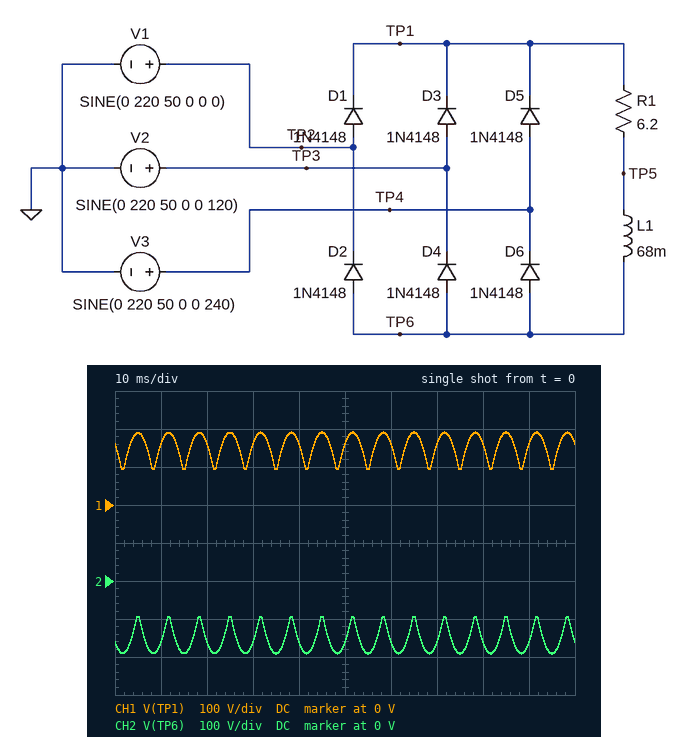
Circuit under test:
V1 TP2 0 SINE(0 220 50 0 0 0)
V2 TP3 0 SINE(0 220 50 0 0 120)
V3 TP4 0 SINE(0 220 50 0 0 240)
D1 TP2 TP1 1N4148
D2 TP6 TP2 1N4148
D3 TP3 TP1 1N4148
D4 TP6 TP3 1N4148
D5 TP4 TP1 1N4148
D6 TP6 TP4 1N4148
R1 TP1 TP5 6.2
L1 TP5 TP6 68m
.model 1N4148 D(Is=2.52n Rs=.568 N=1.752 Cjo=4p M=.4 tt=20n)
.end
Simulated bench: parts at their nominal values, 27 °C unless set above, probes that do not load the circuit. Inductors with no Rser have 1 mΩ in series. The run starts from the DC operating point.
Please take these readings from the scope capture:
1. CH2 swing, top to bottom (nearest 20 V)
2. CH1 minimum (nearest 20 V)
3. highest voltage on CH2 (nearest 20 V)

100 V
100 V
-100 V
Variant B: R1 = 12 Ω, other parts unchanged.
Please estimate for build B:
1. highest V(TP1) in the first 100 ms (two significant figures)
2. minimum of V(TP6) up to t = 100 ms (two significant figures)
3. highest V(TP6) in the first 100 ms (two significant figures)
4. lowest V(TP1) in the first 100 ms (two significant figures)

200 V
-200 V
-100 V
100 V
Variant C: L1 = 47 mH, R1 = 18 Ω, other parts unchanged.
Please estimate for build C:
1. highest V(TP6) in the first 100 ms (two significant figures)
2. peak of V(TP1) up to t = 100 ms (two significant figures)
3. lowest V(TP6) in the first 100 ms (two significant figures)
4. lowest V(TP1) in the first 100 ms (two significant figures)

-100 V
210 V
-210 V
100 V
